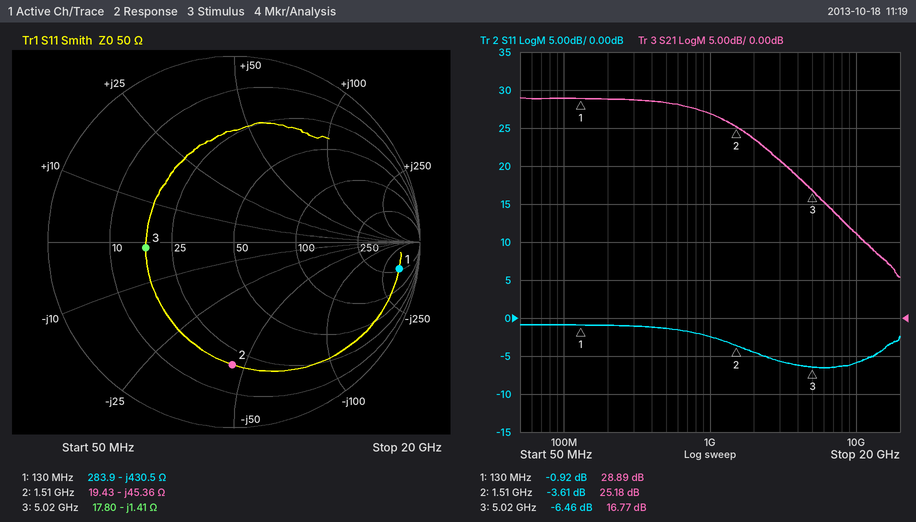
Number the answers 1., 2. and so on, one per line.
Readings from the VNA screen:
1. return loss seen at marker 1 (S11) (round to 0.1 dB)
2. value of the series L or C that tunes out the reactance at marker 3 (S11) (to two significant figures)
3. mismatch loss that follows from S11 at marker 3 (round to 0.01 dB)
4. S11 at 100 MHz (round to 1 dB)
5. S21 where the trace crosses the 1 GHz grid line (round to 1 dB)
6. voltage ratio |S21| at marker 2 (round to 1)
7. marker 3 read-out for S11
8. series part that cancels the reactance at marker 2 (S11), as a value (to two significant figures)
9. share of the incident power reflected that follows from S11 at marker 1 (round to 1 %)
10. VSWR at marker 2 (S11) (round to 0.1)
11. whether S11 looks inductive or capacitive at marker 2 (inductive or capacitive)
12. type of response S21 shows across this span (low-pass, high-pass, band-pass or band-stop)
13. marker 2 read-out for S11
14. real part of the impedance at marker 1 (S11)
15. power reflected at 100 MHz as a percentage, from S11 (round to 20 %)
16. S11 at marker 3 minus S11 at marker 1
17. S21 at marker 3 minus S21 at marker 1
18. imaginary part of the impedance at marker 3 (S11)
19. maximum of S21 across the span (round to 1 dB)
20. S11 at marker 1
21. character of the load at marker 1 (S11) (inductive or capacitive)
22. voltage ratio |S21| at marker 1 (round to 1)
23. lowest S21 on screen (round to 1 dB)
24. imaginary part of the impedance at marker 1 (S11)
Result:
1. 0.9 dB
2. 45 pH
3. 1.11 dB
4. -1 dB
5. 27 dB
6. 18
7. -6.46 dB
8. 4.8 nH
9. 81 %
10. 4.9
11. capacitive
12. low-pass
13. -3.61 dB
14. 283.9 Ω
15. 80 %
16. -5.54 dB
17. -12.12 dB
18. -1.41 Ω
19. 29 dB
20. -0.92 dB
21. capacitive
22. 28
23. 5 dB
24. -430.5 Ω
